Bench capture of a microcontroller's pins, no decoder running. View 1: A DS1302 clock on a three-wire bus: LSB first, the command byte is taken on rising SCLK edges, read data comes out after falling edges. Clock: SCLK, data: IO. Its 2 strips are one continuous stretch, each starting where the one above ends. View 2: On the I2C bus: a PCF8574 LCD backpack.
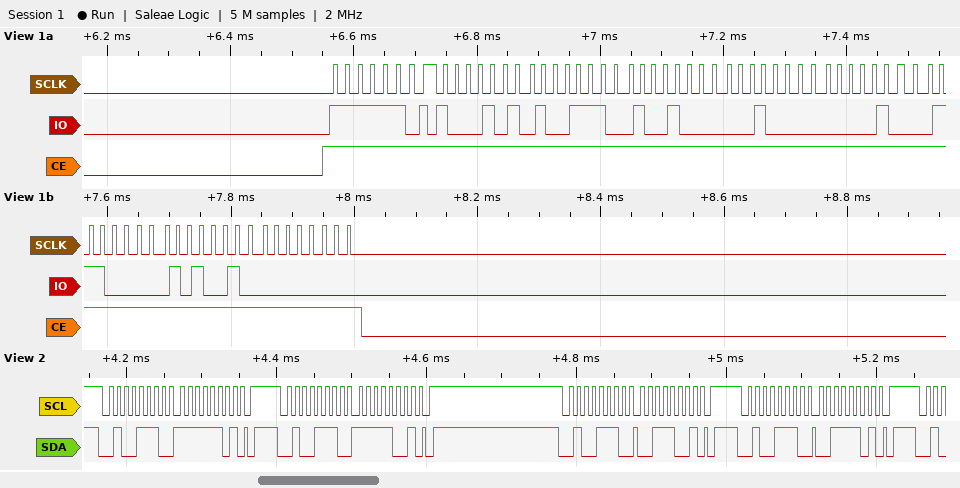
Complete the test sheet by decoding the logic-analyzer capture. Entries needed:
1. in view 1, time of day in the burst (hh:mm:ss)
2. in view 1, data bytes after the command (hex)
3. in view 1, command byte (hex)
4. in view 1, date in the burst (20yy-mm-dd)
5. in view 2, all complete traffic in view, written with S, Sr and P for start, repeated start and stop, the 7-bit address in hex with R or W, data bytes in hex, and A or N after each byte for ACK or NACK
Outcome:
09:39:51
51 39 09 04 10 07 25 00
0xBF
2025-10-04
S 27W A FD A P S 27W A F9 A P S 27W A 39 A P S 27W A 3D A P
